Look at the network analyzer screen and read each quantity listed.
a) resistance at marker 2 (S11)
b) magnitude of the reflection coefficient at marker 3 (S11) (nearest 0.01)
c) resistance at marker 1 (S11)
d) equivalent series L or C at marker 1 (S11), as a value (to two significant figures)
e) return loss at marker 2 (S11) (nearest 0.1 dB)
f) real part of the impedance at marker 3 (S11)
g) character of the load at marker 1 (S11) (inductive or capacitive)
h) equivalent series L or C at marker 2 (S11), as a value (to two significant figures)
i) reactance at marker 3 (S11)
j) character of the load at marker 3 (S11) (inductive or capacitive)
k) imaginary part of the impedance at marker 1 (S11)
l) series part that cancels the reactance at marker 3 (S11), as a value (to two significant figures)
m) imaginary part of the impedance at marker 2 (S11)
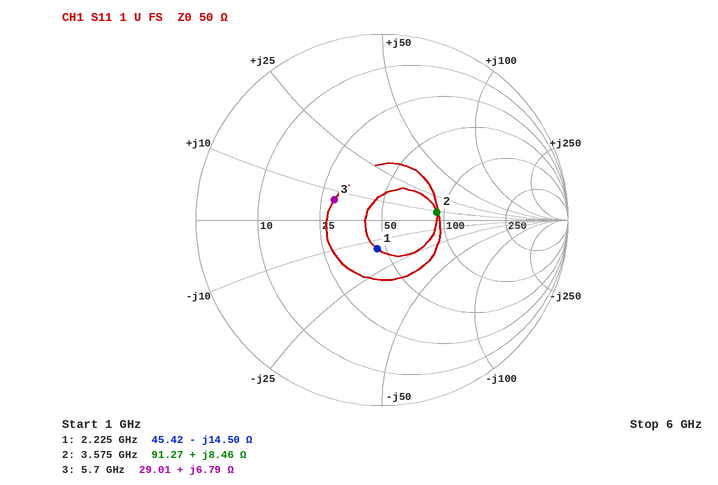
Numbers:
91.27 Ω
0.28
45.42 Ω
4.9 pF
10.5 dB
29.01 Ω
capacitive
380 pH
+6.79 Ω
inductive
-14.50 Ω
4.1 pF
+8.46 Ω
